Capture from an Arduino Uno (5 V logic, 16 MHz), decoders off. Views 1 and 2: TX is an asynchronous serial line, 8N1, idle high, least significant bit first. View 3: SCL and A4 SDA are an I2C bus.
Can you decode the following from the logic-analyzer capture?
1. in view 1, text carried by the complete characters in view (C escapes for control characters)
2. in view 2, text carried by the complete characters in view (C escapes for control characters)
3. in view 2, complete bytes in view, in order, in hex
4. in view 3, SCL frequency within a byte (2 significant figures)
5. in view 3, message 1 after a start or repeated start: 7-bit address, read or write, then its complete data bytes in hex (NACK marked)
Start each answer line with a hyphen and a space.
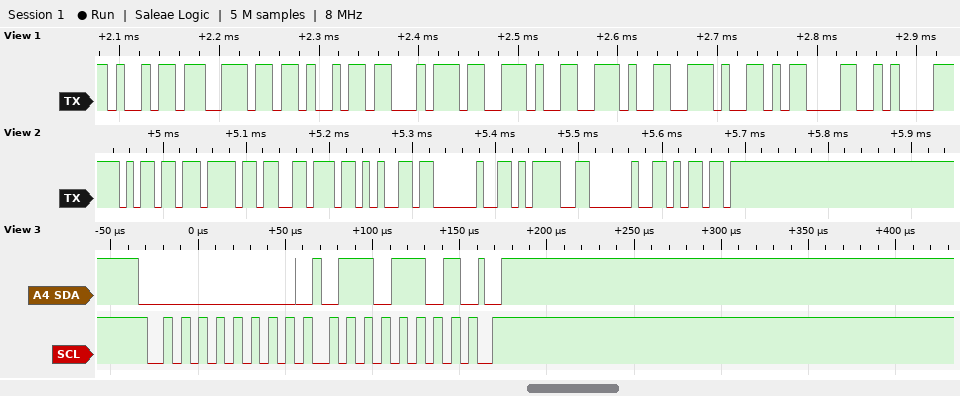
- "init...\r\n"
- "move = m"
- 6D 6F 76 65 20 3D 20 6D
- 100 kHz
- 0x00 write: 6D
